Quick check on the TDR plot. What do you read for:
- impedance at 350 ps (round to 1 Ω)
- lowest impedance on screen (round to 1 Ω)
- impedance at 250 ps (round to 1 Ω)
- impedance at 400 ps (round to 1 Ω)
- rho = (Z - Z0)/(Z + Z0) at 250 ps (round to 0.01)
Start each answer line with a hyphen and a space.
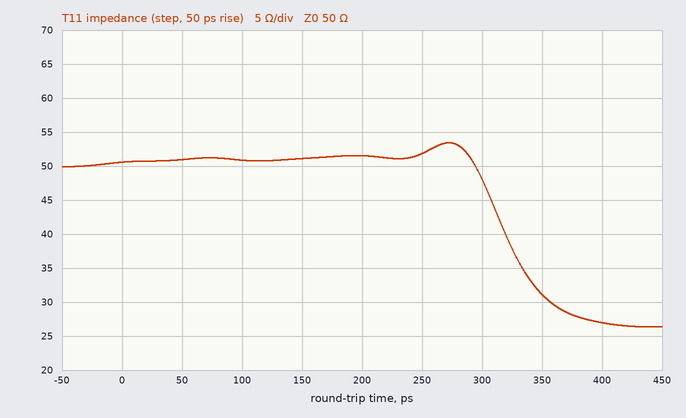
- 31 Ω
- 26 Ω
- 52 Ω
- 27 Ω
- +0.02
